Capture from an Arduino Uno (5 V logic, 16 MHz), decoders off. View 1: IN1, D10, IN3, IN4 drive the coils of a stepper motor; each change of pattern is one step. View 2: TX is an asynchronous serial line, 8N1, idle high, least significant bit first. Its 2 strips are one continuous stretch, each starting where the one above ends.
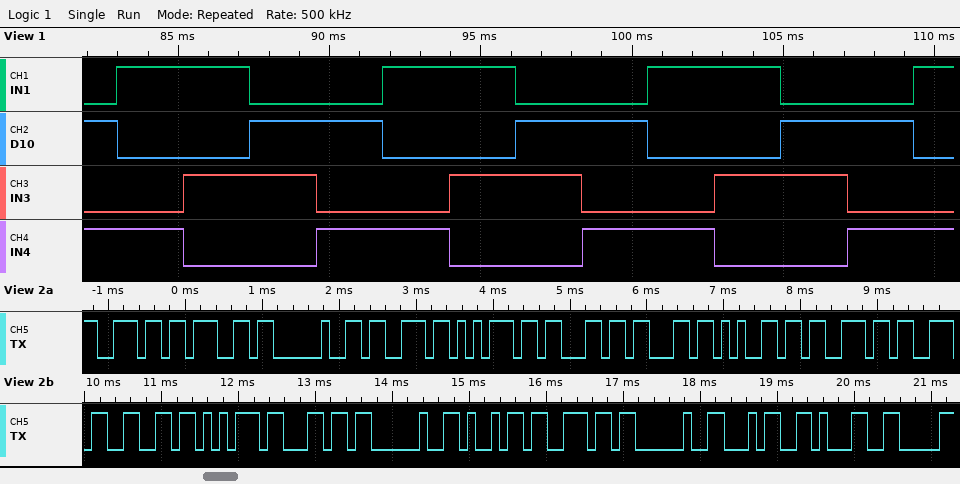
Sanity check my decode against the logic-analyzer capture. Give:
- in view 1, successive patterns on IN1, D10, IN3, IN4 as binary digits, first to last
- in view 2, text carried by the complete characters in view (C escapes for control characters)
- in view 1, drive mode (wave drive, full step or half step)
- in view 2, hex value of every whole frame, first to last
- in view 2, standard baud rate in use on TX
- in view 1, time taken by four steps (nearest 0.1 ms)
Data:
0101 1001 1010 0110 0101 1001 1010 0110 0101 1001 1010 0110 0101 1001
"ng successful in 41"
full step
6E 67 20 73 75 63 63 65 73 73 66 75 6C 20 69 6E 20 34 31
9600 baud
8.8 ms
